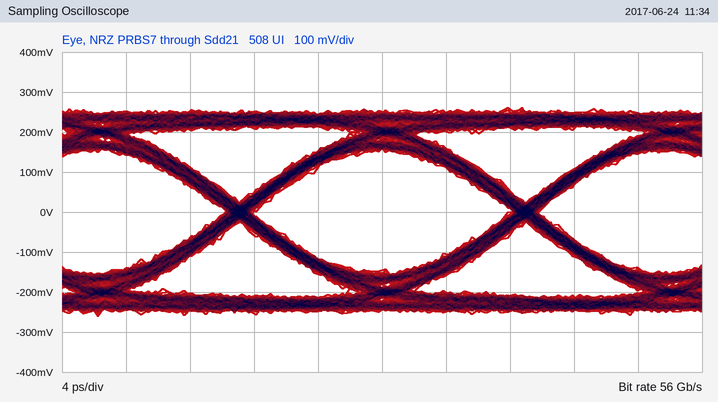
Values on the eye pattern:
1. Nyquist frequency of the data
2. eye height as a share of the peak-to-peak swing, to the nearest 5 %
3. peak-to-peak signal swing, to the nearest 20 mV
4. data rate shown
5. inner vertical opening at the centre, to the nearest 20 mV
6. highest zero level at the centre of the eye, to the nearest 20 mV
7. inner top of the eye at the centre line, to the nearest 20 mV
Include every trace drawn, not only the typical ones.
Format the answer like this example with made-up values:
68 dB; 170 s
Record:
28 GHz; 60 %; 520 mV; 56 Gb/s; 300 mV; -140 mV; 160 mV
